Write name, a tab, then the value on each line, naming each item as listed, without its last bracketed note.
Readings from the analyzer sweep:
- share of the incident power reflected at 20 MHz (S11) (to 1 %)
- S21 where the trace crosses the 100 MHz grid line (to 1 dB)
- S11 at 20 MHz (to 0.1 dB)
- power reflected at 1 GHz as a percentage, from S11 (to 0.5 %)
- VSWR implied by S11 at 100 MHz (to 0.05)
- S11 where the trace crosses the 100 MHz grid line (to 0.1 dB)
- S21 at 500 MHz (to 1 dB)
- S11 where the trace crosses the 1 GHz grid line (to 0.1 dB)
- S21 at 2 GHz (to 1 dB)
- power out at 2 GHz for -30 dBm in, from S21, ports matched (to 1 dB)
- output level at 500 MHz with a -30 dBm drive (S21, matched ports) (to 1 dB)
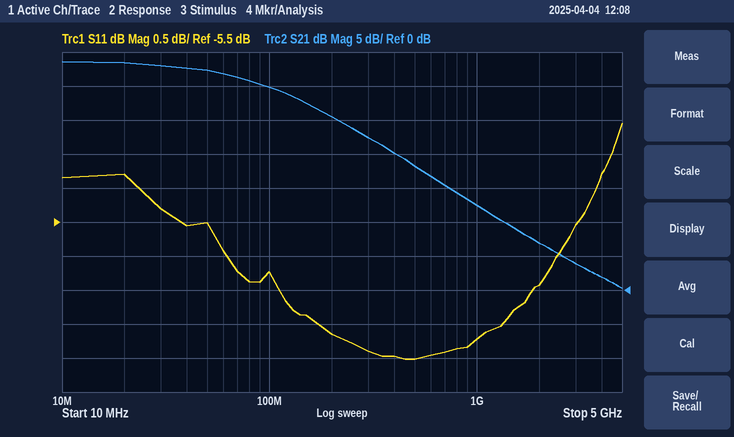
share of the incident power reflected at 20 MHz (S11)	33 %
S21 where the trace crosses the 100 MHz grid line	30 dB
S11 at 20 MHz	-4.8 dB
power reflected at 1 GHz as a percentage, from S11	19.0 %
VSWR implied by S11 at 100 MHz	2.90
S11 where the trace crosses the 100 MHz grid line	-6.2 dB
S21 at 500 MHz	18 dB
S11 where the trace crosses the 1 GHz grid line	-7.2 dB
S21 at 2 GHz	7 dB
power out at 2 GHz for -30 dBm in, from S21, ports matched	-23 dBm
output level at 500 MHz with a -30 dBm drive (S21, matched ports)	-12 dBm
